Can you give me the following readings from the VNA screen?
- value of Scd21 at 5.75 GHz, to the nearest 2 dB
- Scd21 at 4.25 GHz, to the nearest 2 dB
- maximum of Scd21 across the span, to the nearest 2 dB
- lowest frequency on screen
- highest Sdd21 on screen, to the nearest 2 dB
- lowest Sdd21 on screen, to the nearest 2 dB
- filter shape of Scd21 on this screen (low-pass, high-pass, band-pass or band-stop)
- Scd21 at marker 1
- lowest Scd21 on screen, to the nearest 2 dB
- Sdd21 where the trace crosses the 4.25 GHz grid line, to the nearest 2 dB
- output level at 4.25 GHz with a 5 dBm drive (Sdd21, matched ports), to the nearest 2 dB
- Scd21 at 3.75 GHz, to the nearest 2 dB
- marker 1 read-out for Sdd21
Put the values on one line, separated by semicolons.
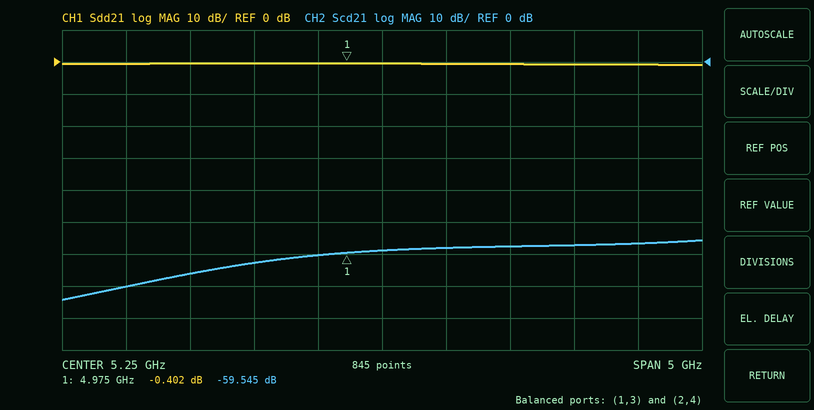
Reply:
-58 dB; -62 dB; -56 dB; 2.75 GHz; 0 dB; 0 dB; high-pass; -59.545 dB; -74 dB; 0 dB; 4 dBm; -66 dB; -0.402 dB
